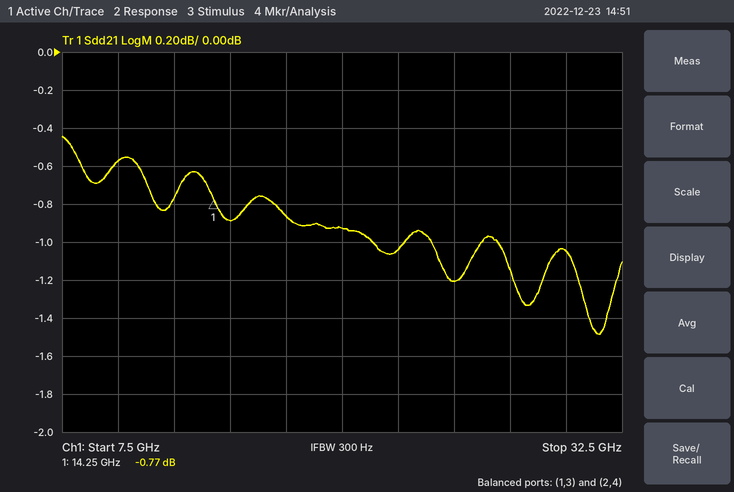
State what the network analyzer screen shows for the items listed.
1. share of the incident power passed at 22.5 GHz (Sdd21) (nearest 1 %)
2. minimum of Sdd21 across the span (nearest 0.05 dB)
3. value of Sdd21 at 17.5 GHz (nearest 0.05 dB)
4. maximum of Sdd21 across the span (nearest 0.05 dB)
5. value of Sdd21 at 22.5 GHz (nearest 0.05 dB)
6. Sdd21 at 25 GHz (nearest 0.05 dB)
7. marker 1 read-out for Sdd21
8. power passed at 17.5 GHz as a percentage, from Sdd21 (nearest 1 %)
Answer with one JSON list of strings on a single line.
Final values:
["79 %", "-1.50 dB", "-0.85 dB", "-0.45 dB", "-1.05 dB", "-1.20 dB", "-0.77 dB", "82 %"]
